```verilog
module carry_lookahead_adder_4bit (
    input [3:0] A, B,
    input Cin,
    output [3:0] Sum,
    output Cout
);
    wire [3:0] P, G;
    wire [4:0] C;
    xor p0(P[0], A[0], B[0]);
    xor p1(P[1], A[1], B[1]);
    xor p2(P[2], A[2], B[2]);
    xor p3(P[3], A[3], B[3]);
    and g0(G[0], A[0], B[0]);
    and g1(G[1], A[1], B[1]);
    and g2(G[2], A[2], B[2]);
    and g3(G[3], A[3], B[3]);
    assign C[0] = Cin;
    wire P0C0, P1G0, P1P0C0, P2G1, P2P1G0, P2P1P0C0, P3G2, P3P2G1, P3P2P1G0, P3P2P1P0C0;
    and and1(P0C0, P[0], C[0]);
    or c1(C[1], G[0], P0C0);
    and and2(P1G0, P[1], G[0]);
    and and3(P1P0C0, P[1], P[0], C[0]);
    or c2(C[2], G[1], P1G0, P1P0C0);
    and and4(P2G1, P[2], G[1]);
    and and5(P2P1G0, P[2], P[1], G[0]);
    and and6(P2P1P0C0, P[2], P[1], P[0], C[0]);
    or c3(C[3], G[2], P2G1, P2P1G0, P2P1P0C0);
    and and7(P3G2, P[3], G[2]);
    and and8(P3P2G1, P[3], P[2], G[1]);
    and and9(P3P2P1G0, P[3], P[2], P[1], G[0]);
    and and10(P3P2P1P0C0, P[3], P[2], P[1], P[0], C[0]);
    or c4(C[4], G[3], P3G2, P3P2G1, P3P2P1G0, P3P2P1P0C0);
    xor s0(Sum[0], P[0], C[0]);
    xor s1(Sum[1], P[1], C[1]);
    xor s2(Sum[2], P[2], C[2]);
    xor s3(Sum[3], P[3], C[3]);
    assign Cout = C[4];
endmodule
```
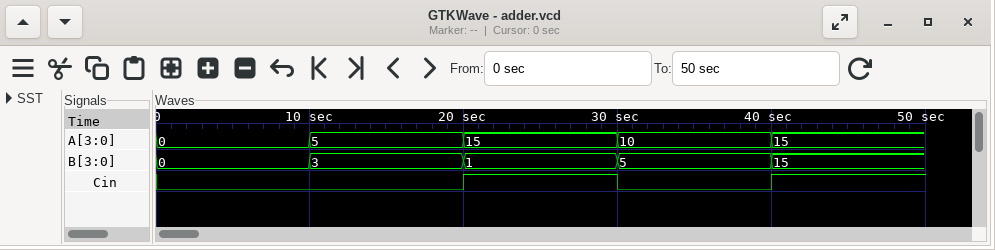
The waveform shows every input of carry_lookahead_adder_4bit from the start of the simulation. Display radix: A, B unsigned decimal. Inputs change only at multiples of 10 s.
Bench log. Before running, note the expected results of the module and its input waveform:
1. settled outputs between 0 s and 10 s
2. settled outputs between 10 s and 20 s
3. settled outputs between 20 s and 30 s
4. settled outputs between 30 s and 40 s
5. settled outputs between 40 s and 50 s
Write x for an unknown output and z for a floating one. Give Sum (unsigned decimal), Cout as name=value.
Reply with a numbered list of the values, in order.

1. Sum=0, Cout=0
2. Sum=8, Cout=0
3. Sum=1, Cout=1
4. Sum=15, Cout=0
5. Sum=15, Cout=1
